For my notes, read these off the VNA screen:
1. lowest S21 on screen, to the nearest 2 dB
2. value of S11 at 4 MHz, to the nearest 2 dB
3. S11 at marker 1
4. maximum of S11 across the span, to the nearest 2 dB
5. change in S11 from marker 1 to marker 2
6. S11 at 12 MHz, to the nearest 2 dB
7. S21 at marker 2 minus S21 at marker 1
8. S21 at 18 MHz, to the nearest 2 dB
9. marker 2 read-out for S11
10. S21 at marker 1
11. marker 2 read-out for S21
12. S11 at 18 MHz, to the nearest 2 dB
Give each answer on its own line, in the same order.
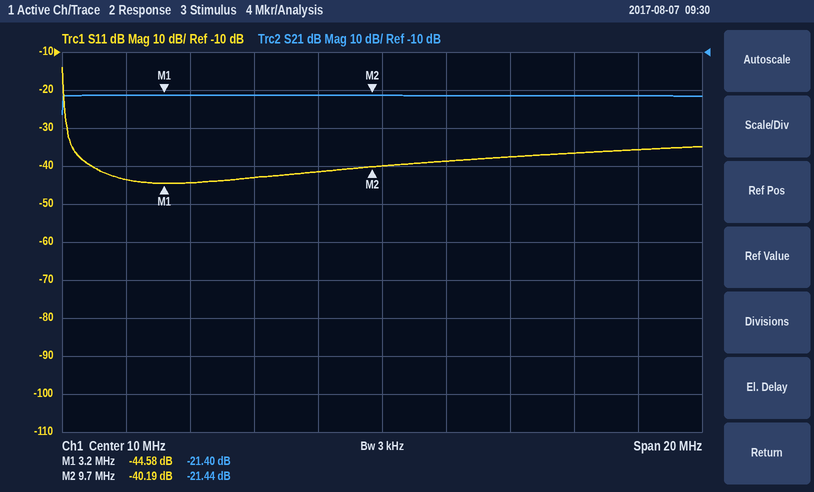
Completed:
-26 dB
-44 dB
-44.58 dB
-14 dB
4.39 dB
-38 dB
-0.04 dB
-22 dB
-40.19 dB
-21.40 dB
-21.44 dB
-36 dB
